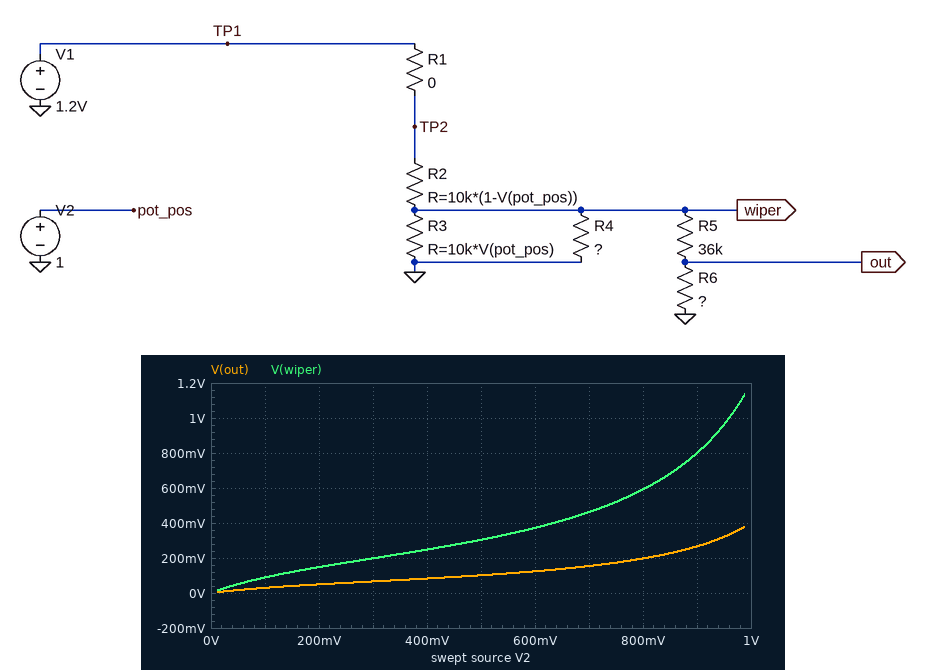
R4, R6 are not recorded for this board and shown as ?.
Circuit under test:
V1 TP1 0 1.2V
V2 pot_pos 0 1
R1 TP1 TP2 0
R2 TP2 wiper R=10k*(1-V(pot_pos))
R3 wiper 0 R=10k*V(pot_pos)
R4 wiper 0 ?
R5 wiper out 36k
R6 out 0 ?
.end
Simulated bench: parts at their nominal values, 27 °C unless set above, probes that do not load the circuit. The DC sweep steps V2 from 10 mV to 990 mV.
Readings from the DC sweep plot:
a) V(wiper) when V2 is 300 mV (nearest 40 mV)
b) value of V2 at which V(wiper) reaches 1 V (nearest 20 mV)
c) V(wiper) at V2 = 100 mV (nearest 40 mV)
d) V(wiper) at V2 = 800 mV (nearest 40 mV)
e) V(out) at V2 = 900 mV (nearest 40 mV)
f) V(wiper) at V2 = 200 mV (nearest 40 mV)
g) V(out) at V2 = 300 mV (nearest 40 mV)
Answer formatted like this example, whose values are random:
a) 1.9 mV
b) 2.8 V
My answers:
a) 200 mV
b) 960 mV
c) 80 mV
d) 600 mV
e) 280 mV
f) 160 mV
g) 80 mV
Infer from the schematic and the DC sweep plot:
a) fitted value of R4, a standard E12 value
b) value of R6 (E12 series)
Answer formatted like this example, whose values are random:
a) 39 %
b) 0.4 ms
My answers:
a) 2.7 kΩ
b) 18 kΩ
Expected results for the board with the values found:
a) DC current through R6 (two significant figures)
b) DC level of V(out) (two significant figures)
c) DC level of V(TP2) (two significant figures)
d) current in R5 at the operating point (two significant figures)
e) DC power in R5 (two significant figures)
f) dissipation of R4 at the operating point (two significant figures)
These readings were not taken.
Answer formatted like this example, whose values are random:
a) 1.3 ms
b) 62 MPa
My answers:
a) 22 µA
b) 400 mV
c) 1.2 V
d) 22 µA
e) 18 µW
f) 530 µW
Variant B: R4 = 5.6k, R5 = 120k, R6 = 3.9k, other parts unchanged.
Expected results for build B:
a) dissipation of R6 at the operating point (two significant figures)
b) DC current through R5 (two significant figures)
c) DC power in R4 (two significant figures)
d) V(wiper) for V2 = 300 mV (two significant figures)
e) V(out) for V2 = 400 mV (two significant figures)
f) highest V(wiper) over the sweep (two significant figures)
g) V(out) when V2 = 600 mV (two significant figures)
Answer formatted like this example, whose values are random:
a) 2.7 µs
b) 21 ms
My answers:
a) 370 nW
b) 9.7 µA
c) 260 µW
d) 260 mV
e) 10 mV
f) 1.2 V
g) 16 mV
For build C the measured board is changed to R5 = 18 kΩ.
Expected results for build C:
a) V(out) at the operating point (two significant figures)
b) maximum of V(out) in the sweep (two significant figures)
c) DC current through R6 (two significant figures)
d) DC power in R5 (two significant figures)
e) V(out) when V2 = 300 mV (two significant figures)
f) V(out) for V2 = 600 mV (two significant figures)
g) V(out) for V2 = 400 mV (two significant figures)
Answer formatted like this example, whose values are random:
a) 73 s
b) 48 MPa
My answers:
a) 600 mV
b) 570 mV
c) 33 µA
d) 20 µW
e) 98 mV
f) 180 mV
g) 120 mV
